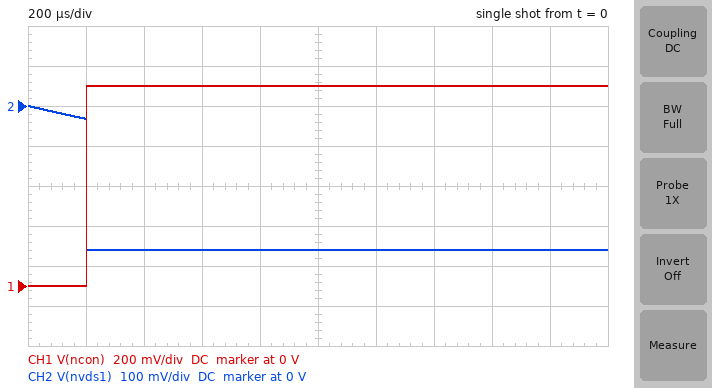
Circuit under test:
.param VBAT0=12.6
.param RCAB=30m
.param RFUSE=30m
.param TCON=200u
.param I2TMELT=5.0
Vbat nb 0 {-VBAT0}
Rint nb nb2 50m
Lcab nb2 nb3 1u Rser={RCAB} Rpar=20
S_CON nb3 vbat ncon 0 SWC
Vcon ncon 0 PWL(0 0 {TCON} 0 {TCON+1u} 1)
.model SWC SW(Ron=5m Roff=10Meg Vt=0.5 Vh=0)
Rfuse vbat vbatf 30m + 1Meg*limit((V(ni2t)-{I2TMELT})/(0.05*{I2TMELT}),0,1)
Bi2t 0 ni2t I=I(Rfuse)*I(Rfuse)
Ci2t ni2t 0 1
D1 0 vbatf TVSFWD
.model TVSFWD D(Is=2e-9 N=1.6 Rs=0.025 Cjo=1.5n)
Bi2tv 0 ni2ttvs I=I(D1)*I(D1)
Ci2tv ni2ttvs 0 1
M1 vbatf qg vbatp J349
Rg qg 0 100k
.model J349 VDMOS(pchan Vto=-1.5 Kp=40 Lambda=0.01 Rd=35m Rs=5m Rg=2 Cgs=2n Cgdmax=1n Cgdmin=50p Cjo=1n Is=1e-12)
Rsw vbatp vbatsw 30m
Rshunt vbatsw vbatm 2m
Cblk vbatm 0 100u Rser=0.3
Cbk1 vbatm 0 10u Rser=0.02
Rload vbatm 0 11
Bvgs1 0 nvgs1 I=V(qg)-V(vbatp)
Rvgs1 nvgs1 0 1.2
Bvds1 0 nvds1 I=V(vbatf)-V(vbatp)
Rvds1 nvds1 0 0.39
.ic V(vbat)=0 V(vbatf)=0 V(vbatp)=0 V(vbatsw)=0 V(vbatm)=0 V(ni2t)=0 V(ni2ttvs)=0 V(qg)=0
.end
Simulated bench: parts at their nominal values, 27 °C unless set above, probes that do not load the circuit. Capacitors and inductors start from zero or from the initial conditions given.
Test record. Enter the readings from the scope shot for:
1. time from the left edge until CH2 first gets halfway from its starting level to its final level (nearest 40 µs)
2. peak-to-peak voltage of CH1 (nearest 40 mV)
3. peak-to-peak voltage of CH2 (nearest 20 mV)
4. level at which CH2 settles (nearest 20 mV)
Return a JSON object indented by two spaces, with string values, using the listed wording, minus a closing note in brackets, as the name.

{
  "time from the left edge until CH2 first gets halfway from its starting level to its final level": "200 µs",
  "peak-to-peak voltage of CH1": "1.00 V",
  "peak-to-peak voltage of CH2": "360 mV",
  "level at which CH2 settles": "-360 mV"
}
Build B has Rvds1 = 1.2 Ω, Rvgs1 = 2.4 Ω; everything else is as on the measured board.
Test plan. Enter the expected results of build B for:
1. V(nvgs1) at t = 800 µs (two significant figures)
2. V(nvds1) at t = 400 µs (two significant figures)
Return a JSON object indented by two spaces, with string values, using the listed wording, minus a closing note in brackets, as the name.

{
  "V(nvgs1) at t = 800 µs": "-34 mV",
  "V(nvds1) at t = 400 µs": "-1.1 V"
}
